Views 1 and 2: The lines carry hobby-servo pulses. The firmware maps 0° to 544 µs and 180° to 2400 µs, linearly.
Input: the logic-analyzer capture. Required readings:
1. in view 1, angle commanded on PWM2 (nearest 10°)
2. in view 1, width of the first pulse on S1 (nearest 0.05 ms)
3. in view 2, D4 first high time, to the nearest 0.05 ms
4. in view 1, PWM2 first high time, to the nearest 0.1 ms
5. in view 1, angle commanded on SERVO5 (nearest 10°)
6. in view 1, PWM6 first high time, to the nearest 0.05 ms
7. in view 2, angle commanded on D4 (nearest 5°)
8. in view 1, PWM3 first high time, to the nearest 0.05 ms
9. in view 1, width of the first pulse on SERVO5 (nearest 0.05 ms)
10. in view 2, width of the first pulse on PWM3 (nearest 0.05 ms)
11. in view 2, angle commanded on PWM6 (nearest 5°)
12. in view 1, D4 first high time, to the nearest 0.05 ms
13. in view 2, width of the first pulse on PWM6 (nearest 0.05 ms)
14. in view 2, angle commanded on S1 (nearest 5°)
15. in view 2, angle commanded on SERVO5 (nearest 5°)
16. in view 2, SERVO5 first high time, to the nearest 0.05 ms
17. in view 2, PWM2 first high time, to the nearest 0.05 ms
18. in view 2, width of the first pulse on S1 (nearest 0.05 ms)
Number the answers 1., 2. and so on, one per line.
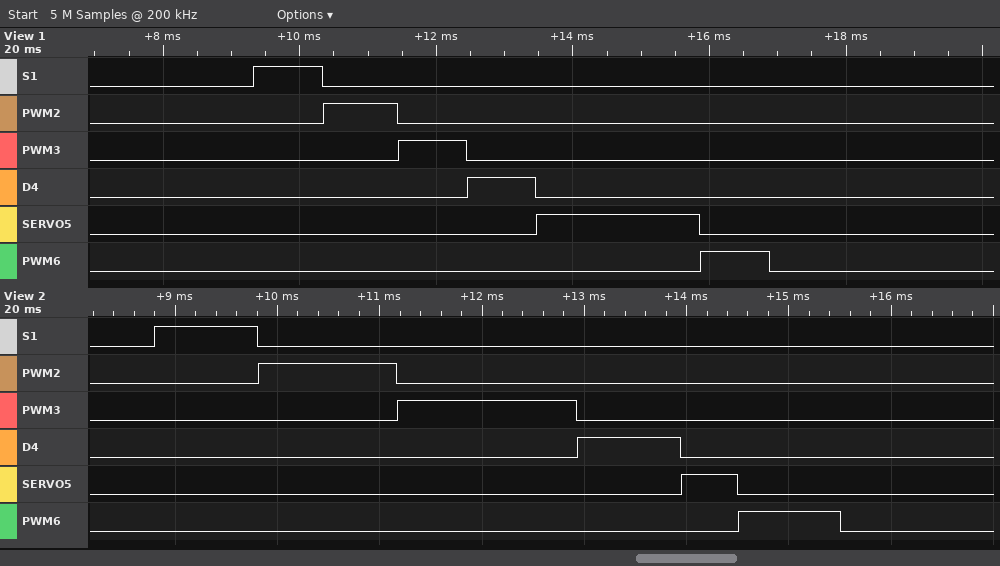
1. 50°
2. 1.00 ms
3. 1.00 ms
4. 1.1 ms
5. 180°
6. 1.00 ms
7. 45°
8. 1.00 ms
9. 2.40 ms
10. 1.75 ms
11. 45°
12. 1.00 ms
13. 1.00 ms
14. 45°
15. 0°
16. 0.55 ms
17. 1.35 ms
18. 1.00 ms
